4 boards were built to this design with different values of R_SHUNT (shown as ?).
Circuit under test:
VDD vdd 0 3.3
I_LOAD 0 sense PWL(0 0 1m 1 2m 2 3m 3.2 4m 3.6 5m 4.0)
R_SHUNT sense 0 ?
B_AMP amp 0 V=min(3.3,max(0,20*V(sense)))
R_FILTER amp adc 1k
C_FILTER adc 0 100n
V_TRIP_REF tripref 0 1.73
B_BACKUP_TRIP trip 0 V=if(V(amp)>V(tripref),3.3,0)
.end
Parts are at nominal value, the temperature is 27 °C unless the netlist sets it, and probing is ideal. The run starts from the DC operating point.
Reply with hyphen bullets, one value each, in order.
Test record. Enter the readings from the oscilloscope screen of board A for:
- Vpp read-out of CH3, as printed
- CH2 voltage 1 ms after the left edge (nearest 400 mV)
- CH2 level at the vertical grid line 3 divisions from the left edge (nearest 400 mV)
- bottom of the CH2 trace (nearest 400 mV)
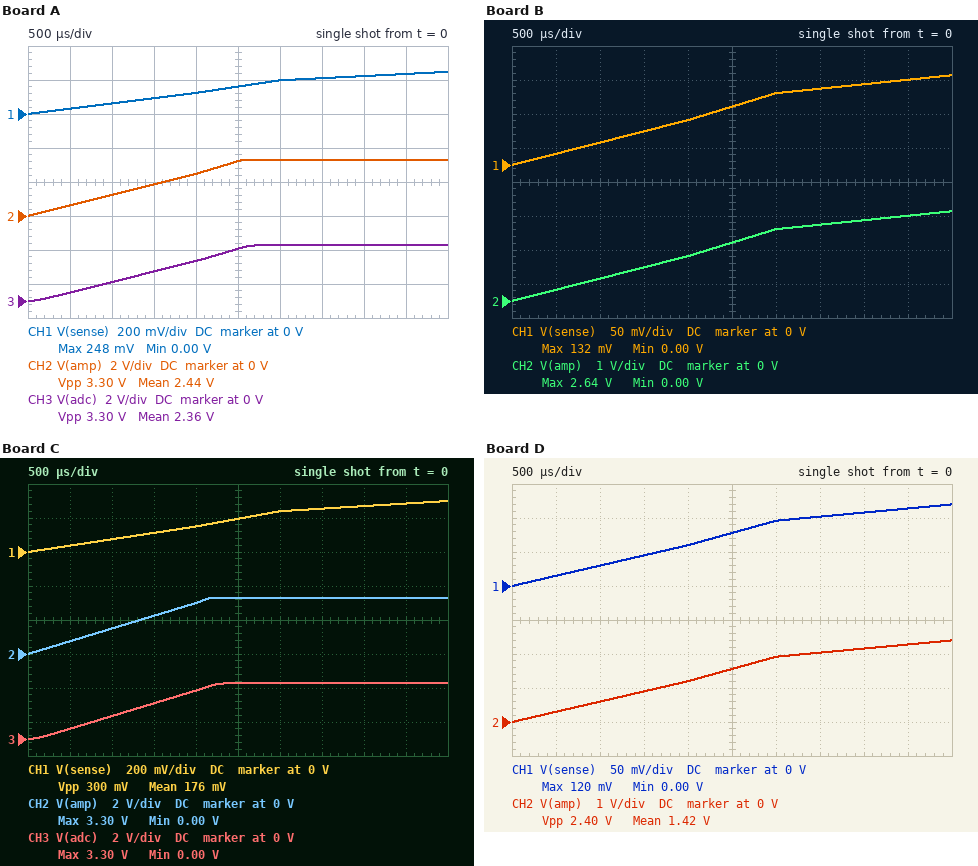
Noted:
- 3.30 V
- 1.2 V
- 2.0 V
- 0 V
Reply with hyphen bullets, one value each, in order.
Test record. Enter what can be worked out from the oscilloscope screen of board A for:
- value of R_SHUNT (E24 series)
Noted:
- 0.062 Ω
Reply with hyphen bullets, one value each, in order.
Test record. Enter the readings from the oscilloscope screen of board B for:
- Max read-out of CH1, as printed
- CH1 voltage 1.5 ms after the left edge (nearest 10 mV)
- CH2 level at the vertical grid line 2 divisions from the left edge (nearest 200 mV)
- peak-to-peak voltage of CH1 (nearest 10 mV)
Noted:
- 132 mV
- 50 mV
- 600 mV
- 130 mV
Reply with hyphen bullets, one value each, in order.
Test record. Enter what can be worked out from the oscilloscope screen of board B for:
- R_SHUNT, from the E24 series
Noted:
- 0.033 Ω
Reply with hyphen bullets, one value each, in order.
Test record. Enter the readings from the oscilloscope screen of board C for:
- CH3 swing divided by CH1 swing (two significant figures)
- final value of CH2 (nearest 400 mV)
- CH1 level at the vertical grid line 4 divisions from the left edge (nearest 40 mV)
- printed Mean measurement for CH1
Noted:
- 11
- 3.2 V
- 160 mV
- 176 mV
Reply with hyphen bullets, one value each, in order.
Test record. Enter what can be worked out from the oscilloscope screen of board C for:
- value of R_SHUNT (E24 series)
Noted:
- 0.075 Ω
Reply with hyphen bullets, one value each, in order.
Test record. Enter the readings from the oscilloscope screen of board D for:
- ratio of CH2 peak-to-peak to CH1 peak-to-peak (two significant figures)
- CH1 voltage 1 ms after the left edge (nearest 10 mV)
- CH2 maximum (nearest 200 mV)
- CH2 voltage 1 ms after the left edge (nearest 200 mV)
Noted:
- 20
- 30 mV
- 2.4 V
- 600 mV
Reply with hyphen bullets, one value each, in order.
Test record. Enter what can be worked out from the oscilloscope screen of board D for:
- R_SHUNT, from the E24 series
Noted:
- 0.03 Ω
